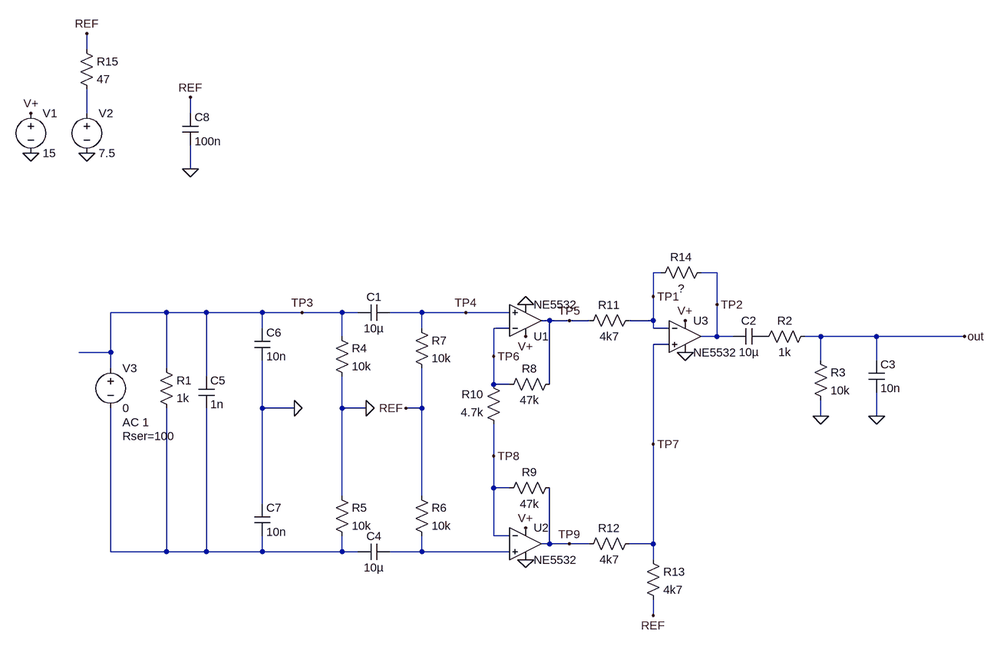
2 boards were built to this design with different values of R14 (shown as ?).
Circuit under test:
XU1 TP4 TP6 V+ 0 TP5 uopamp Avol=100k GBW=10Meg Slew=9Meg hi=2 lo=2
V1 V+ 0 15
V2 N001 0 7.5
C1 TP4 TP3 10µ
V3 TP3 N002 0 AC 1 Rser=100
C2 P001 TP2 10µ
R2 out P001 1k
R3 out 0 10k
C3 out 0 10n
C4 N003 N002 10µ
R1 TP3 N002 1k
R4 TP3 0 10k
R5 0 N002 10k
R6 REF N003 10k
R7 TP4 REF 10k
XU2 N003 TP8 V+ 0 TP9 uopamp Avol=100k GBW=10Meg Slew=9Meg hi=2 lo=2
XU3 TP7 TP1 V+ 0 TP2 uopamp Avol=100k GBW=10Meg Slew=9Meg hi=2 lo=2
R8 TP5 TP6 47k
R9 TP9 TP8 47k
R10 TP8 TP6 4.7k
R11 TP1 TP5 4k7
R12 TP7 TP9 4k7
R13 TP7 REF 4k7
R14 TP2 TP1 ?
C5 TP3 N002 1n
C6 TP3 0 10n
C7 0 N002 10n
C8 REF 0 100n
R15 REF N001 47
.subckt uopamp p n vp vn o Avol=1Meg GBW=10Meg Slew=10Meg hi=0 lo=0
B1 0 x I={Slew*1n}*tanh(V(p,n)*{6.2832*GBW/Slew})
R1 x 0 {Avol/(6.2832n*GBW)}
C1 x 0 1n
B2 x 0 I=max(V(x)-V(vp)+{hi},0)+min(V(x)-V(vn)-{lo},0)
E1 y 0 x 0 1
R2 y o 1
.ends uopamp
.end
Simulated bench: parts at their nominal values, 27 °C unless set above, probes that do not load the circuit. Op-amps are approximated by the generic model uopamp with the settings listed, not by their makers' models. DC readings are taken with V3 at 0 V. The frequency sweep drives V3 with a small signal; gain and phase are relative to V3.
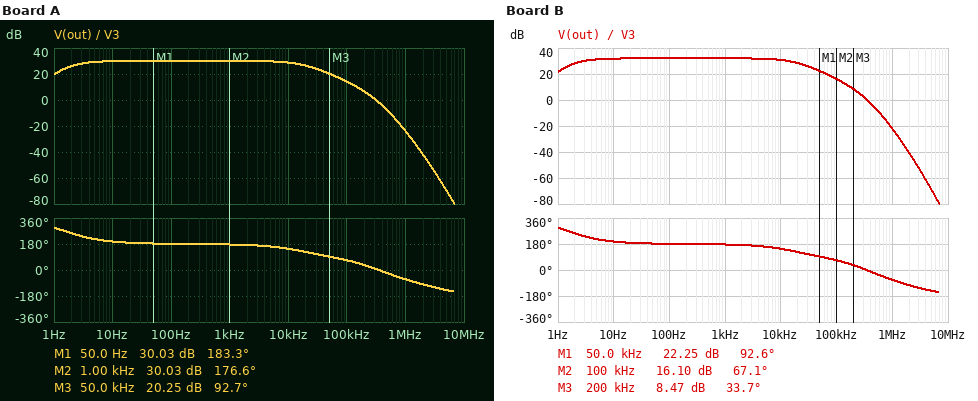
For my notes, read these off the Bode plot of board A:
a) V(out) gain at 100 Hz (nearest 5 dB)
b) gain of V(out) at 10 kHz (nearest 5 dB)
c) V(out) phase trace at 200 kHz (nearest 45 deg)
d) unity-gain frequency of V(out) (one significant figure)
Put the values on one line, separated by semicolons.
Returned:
30 dB; 30 dB; 45 deg; 300 kHz
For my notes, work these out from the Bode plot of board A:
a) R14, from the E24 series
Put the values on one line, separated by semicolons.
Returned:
10 kΩ
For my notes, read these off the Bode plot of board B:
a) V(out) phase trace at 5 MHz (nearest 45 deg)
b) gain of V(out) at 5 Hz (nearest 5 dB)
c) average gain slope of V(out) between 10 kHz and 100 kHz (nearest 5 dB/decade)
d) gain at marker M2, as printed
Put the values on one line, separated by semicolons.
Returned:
-135 deg; 30 dB; -15 dB/decade; 16.10 dB
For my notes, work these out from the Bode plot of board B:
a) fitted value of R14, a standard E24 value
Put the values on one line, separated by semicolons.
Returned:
13 kΩ
